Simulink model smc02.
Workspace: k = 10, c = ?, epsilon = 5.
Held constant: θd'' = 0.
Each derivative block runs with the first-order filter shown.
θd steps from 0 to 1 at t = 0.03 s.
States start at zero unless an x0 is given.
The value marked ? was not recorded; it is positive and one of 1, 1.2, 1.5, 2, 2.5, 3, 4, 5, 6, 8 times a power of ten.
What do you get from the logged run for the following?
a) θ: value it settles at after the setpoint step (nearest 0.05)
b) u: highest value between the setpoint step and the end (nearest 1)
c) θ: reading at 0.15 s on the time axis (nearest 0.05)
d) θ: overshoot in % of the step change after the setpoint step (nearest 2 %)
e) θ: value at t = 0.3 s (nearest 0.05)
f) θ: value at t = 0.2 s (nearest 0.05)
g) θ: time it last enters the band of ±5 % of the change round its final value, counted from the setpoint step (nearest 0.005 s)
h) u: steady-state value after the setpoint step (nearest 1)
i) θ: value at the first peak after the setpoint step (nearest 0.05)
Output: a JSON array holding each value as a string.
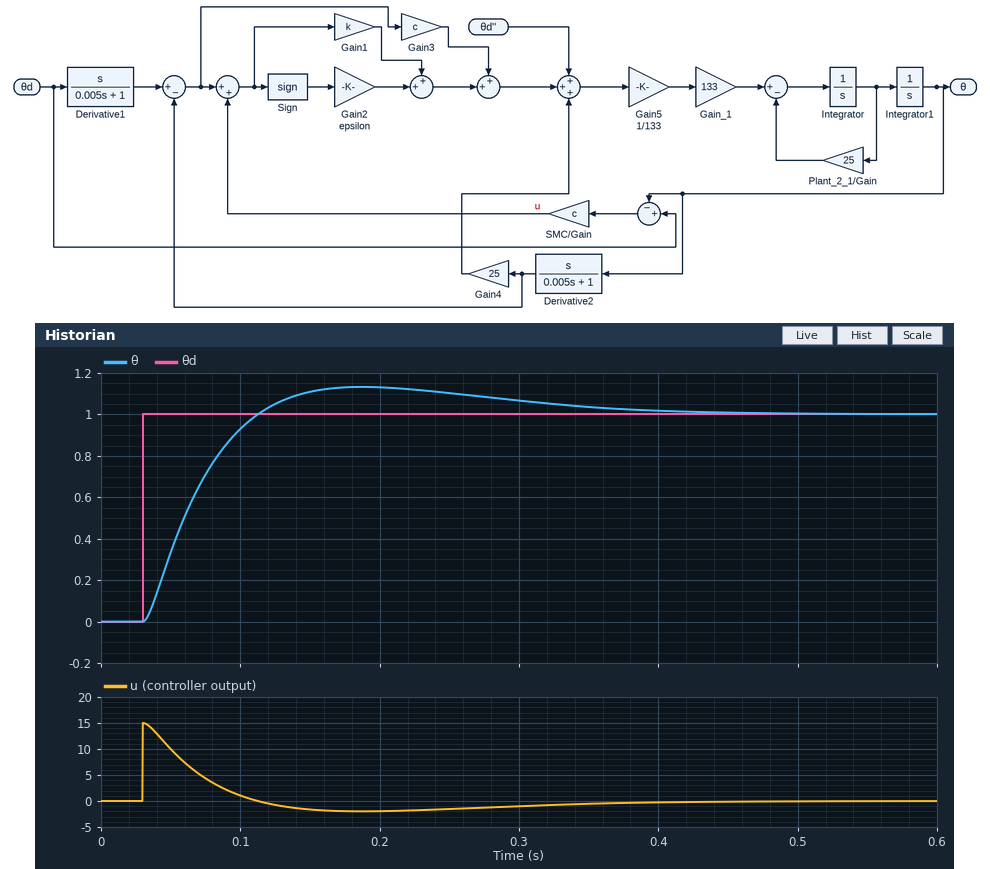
["1.00", "15", "1.10", "14 %", "1.05", "1.15", "0.295 s", "0", "1.15"]
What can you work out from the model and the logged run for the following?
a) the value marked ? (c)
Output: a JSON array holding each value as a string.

["15"]
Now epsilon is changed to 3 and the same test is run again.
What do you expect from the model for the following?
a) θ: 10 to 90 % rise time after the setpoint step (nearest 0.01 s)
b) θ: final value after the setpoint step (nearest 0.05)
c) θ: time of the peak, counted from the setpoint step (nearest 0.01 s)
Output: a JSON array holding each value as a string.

["0.06 s", "1.00", "0.16 s"]
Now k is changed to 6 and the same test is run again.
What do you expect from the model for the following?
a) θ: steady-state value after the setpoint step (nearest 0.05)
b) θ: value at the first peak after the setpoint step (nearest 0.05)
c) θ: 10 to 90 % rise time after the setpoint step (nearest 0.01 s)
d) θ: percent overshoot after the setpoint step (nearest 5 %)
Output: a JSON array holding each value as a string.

["1.00", "1.10", "0.07 s", "10 %"]
